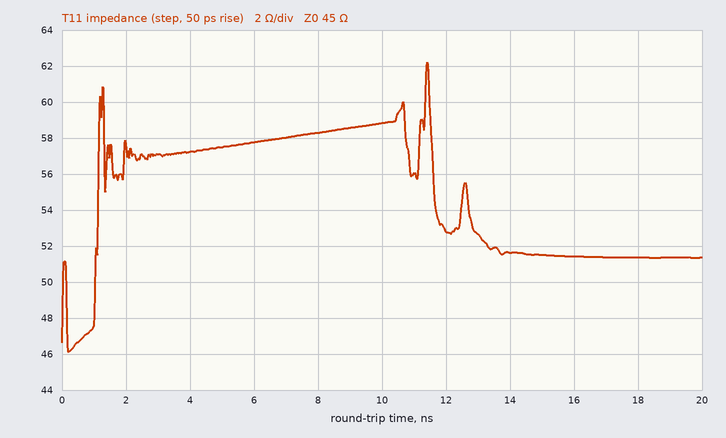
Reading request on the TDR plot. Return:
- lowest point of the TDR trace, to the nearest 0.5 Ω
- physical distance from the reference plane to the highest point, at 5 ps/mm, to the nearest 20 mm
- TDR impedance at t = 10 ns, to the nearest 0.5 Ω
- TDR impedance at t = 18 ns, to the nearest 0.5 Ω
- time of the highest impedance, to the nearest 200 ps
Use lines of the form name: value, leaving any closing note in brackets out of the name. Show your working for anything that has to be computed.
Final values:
lowest point of the TDR trace, to the nearest 0.5 Ω: 46.0 Ω
physical distance from the reference plane to the highest point, at 5 ps/mm, to the nearest 20 mm: 11.4 ns / 2 / 5 ps/mm ≈ 1.14 m
TDR impedance at t = 10 ns, to the nearest 0.5 Ω: 59.0 Ω
TDR impedance at t = 18 ns, to the nearest 0.5 Ω: 51.5 Ω
time of the highest impedance, to the nearest 200 ps: 11.4 ns
